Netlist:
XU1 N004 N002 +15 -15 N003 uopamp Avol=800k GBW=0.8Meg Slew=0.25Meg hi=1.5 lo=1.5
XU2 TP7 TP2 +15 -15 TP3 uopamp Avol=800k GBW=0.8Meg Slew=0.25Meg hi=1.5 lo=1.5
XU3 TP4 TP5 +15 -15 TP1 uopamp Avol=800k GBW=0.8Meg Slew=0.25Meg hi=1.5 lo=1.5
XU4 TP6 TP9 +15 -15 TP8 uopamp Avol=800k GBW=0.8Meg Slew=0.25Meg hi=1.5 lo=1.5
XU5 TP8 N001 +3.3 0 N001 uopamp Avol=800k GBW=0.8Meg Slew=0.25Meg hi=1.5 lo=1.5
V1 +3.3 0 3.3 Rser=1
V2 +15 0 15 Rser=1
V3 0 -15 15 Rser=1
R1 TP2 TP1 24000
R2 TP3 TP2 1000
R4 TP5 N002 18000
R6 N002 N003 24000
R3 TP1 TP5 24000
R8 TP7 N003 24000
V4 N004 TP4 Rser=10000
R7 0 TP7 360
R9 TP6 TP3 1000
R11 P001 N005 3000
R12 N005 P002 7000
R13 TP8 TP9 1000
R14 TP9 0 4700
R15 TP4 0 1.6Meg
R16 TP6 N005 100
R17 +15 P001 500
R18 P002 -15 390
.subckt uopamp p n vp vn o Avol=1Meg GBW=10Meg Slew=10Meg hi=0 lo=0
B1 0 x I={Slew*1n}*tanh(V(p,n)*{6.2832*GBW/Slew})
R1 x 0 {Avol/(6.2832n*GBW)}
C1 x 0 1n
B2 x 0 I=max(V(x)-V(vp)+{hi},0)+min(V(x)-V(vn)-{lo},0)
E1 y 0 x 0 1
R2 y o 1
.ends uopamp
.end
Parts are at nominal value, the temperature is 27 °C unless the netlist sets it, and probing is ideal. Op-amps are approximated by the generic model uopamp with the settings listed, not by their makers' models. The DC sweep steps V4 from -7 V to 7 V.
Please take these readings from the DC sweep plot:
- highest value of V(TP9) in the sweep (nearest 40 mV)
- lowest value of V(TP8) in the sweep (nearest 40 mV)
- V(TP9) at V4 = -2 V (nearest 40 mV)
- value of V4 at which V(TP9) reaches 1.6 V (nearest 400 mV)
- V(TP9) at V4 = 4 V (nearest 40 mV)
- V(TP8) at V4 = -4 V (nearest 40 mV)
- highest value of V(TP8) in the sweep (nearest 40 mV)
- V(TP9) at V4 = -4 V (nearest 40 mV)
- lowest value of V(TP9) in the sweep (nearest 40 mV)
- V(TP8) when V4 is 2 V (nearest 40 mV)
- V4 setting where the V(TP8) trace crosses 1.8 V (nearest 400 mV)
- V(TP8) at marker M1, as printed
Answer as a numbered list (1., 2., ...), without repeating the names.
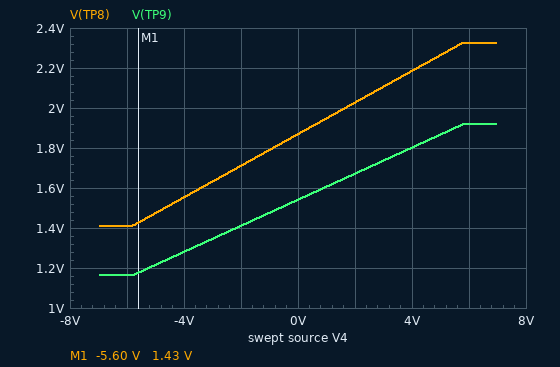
1. 1.92 V
2. 1.40 V
3. 1.40 V
4. 800 mV
5. 1.80 V
6. 1.56 V
7. 2.32 V
8. 1.28 V
9. 1.16 V
10. 2.04 V
11. -800 mV
12. 1.43 V
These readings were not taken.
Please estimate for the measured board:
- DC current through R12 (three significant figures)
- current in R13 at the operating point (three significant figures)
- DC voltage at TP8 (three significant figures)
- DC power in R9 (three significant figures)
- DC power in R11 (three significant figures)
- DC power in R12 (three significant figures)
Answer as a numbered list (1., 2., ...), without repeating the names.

1. 2.26 mA
2. 328 µA
3. 1.87 V
4. 2.38 mW
5. 43.3 mW
6. 35.7 mW
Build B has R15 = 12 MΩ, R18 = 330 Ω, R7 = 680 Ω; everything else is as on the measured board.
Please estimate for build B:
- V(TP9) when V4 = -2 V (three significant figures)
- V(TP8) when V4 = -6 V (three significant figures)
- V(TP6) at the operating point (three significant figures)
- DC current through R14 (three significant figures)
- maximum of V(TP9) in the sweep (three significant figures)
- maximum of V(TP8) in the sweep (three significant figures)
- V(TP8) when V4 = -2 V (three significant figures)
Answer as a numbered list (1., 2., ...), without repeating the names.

1. 1.35 V
2. 1.24 V
3. 1.53 V
4. 325 µA
5. 2.03 V
6. 2.47 V
7. 1.64 V
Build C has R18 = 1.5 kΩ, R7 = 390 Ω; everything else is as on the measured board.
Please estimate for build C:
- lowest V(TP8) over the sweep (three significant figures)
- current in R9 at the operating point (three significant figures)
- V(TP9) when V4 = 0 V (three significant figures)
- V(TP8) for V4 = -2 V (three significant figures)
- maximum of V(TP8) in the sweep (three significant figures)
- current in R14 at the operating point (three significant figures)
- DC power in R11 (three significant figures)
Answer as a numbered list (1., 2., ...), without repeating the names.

1. 1.64 V
2. 1.75 mA
3. 1.75 V
4. 1.95 V
5. 2.59 V
6. 371 µA
7. 41.9 mW
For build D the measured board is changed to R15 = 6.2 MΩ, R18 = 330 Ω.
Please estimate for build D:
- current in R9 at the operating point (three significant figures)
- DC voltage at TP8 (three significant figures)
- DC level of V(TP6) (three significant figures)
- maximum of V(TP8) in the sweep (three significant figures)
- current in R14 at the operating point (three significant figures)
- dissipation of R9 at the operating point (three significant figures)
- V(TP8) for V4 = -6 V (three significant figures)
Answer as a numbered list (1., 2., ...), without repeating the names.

1. 1.53 mA
2. 1.85 V
3. 1.53 V
4. 2.31 V
5. 325 µA
6. 2.34 mW
7. 1.40 V
